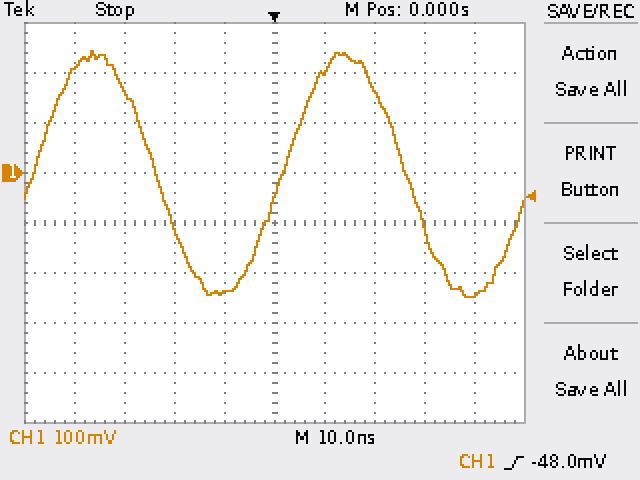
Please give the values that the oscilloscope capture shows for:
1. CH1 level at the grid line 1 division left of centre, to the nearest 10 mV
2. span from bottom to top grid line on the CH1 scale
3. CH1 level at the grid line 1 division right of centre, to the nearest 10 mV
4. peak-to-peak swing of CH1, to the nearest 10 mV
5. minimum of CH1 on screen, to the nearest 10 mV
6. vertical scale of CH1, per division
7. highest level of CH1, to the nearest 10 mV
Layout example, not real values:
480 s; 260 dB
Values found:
-240 mV; 800 mV; 200 mV; 490 mV; -250 mV; 100 mV; 240 mV
